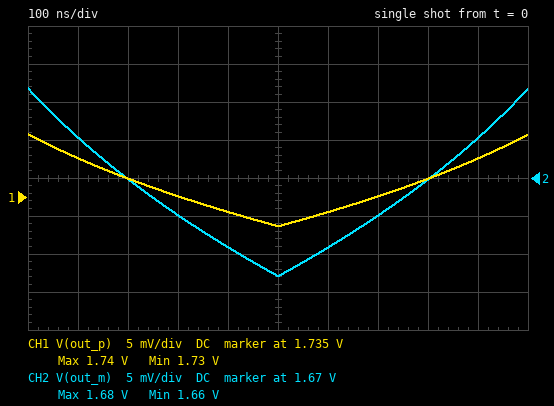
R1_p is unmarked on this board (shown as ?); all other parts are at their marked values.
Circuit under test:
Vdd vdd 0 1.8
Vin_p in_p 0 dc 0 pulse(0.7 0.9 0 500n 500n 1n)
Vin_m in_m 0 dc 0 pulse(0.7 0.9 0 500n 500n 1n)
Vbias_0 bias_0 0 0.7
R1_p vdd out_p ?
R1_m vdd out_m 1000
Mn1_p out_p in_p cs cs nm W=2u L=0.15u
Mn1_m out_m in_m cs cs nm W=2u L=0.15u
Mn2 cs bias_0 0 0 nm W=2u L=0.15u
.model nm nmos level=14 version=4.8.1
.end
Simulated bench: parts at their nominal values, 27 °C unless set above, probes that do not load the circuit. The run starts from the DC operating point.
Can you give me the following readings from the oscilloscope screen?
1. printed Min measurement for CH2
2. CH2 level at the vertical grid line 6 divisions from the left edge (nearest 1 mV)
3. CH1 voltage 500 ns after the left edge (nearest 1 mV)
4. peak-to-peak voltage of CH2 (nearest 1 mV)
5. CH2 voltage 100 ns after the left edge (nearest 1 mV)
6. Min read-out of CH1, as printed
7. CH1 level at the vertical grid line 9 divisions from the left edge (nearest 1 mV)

1.66 V
1.661 V
1.731 V
25 mV
1.675 V
1.73 V
1.740 V
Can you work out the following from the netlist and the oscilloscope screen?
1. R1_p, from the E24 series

470 Ω
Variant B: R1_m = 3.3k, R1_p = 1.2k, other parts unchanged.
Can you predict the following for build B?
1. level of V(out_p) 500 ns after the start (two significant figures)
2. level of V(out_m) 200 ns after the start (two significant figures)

1.6 V
1.4 V
